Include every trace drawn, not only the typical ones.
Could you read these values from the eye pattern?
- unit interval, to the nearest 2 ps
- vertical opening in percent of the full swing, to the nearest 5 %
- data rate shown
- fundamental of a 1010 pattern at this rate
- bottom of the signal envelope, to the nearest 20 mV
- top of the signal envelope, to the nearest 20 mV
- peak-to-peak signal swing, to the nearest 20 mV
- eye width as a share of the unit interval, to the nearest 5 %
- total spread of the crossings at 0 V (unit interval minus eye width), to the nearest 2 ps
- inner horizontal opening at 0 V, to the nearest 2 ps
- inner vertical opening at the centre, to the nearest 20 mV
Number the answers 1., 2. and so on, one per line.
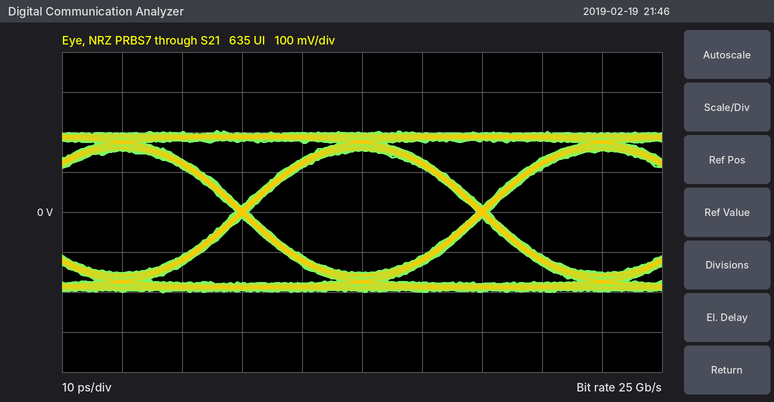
1. 40 ps
2. 75 %
3. 25 Gb/s
4. 12.5 GHz
5. -200 mV
6. 200 mV
7. 400 mV
8. 95 %
9. 2 ps
10. 38 ps
11. 300 mV
